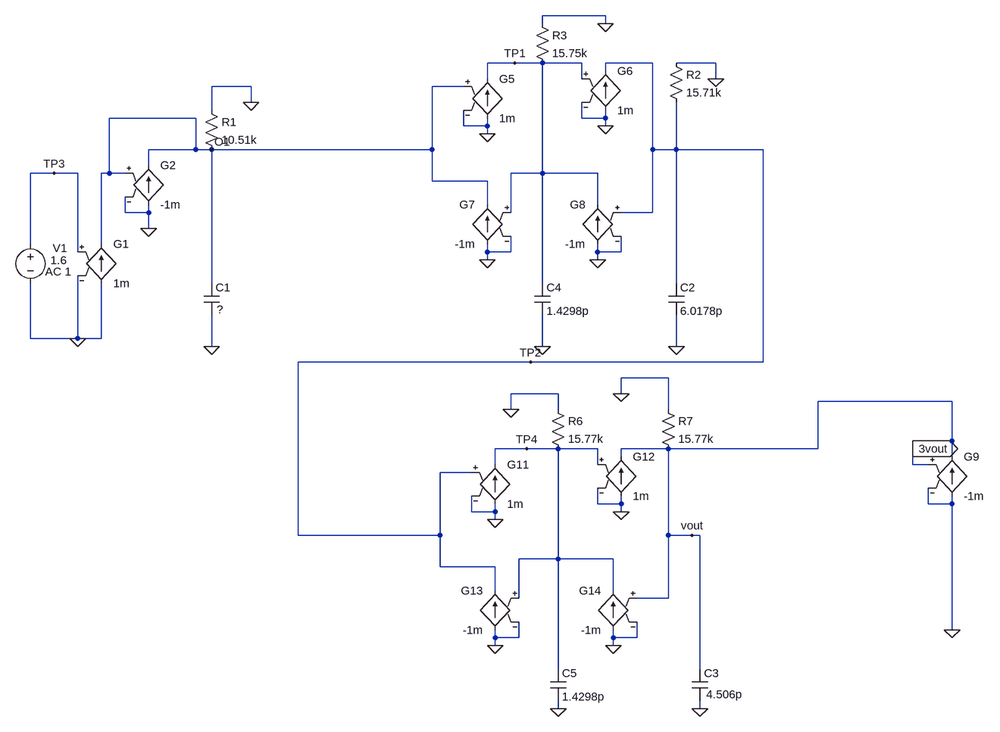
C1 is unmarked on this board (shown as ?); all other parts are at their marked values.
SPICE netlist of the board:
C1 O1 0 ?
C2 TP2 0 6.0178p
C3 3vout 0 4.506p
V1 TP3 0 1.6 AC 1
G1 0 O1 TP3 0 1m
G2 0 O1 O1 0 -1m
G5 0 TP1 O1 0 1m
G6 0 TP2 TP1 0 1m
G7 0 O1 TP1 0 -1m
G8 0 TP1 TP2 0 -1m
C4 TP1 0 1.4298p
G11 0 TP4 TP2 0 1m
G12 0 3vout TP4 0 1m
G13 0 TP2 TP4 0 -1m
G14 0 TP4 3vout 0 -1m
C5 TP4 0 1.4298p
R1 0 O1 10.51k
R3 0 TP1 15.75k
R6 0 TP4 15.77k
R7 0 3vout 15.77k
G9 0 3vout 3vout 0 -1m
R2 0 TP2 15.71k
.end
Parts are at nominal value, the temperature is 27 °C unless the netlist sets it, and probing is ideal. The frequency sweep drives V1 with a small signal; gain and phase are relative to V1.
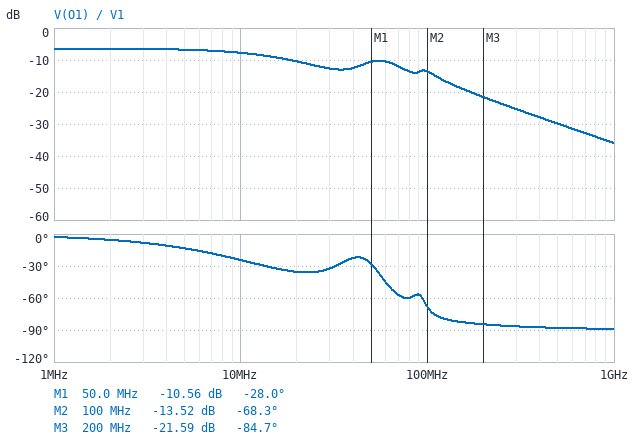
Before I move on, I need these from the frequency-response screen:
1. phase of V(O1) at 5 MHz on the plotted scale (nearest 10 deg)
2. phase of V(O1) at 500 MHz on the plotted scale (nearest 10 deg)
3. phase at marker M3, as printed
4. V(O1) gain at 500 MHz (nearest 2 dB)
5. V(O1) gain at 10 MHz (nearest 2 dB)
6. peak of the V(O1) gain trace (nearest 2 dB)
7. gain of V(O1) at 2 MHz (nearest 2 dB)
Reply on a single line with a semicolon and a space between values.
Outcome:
-10 deg; -90 deg; -84.7 deg; -30 dB; -8 dB; -6 dB; -6 dB
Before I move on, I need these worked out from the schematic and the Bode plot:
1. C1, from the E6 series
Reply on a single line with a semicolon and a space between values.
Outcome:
10 pF
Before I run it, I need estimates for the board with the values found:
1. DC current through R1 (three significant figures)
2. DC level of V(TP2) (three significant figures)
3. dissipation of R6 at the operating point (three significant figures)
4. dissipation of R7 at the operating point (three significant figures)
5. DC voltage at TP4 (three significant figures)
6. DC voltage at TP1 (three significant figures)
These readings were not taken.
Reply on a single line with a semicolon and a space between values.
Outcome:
72.9 µA; 718 mV; 32.4 µW; 28.7 µW; 715 mV; 761 mV
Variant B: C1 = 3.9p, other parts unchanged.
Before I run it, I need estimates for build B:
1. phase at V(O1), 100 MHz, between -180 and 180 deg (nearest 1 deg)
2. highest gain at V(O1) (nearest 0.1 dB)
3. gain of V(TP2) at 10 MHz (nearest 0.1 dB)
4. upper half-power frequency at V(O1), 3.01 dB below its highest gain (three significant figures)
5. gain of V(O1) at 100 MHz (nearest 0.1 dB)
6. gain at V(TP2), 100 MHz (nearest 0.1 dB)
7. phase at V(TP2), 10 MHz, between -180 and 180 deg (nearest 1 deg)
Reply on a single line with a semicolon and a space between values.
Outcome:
-18 deg; -4.8 dB; -7.5 dB; 131 MHz; -5.3 dB; -6.5 dB; -23 deg
